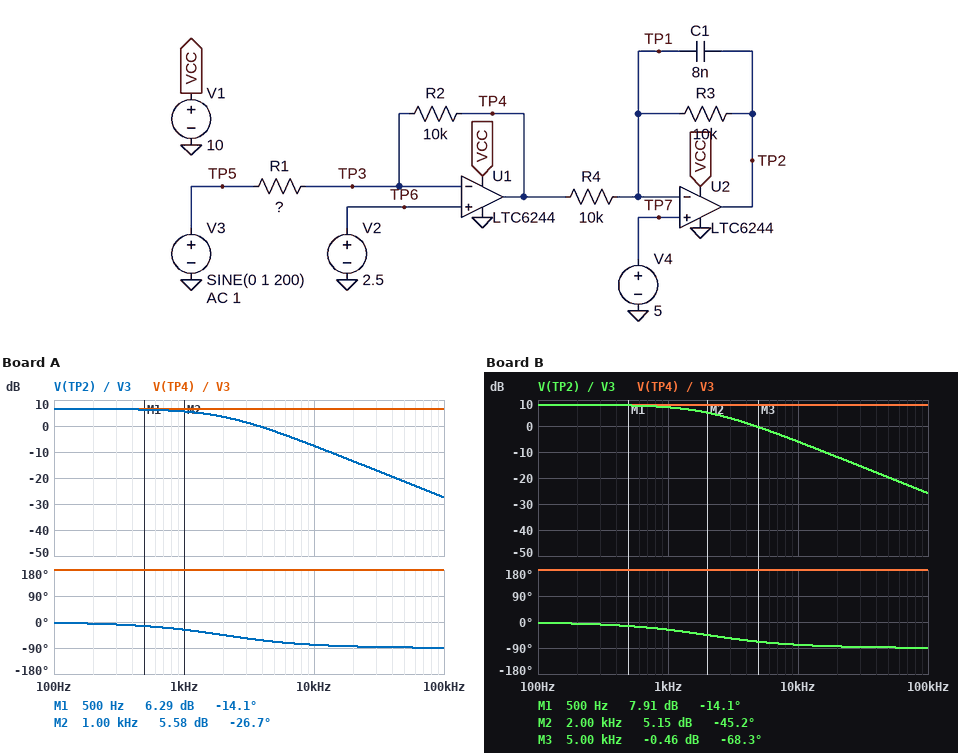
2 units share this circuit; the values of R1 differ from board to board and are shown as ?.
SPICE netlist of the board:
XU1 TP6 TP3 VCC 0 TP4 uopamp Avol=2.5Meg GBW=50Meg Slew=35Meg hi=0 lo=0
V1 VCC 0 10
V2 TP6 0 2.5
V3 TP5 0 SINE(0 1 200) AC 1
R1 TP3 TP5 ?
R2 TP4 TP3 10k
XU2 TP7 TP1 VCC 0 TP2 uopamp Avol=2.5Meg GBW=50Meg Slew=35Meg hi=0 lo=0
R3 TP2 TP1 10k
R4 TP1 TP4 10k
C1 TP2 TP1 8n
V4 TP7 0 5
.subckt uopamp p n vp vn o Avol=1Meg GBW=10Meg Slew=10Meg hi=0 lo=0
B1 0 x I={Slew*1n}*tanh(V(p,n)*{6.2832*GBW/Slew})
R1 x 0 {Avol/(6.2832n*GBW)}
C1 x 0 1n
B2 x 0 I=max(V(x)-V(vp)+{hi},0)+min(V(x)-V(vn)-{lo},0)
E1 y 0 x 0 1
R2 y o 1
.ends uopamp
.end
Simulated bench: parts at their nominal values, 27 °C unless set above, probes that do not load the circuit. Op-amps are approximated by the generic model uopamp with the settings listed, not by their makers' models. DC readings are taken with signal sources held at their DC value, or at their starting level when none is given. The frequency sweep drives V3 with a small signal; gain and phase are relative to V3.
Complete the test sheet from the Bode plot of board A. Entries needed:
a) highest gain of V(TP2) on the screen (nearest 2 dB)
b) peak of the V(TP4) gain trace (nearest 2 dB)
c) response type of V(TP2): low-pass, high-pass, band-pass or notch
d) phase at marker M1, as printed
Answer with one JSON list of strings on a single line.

["6 dB", "6 dB", "low-pass", "-14.1 deg"]
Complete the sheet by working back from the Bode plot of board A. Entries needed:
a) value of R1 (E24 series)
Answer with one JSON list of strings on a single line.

["4.7 kΩ"]
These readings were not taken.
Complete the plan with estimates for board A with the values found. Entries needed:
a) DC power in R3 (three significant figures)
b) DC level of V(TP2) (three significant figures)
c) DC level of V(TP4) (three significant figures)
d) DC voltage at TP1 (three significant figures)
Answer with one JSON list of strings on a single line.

["795 µW", "2.18 V", "7.82 V", "5.00 V"]
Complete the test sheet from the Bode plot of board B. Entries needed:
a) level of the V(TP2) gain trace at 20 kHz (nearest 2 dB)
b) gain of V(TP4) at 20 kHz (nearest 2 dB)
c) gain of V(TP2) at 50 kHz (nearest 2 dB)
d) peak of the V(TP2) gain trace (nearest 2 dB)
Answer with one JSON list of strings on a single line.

["-12 dB", "8 dB", "-20 dB", "8 dB"]
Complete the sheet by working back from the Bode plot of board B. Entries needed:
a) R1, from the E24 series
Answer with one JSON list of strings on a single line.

["3.9 kΩ"]
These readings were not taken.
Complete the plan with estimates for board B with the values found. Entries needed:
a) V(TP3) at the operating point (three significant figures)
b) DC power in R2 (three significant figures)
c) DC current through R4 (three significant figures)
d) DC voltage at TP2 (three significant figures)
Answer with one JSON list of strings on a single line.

["2.50 V", "4.11 mW", "391 µA", "1.09 V"]
